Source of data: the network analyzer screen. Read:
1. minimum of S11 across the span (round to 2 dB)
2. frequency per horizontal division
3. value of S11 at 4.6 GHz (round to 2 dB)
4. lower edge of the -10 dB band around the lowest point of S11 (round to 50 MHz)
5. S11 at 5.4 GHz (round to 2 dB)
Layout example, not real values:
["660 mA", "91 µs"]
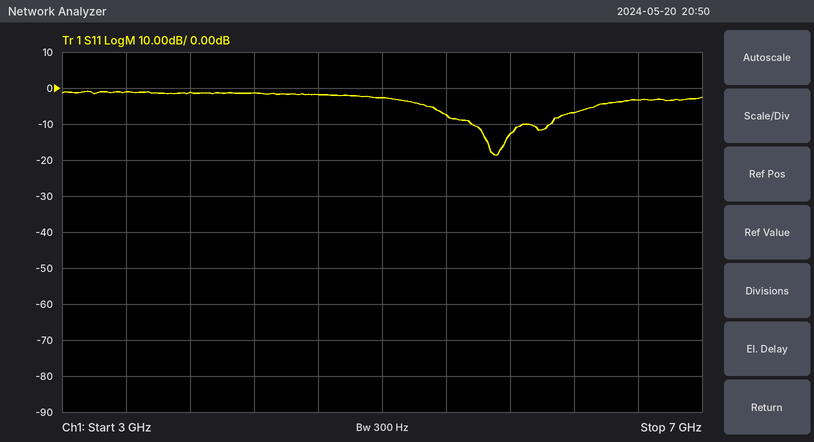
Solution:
["-18 dB", "400 MHz", "-2 dB", "5.55 GHz", "-8 dB"]
